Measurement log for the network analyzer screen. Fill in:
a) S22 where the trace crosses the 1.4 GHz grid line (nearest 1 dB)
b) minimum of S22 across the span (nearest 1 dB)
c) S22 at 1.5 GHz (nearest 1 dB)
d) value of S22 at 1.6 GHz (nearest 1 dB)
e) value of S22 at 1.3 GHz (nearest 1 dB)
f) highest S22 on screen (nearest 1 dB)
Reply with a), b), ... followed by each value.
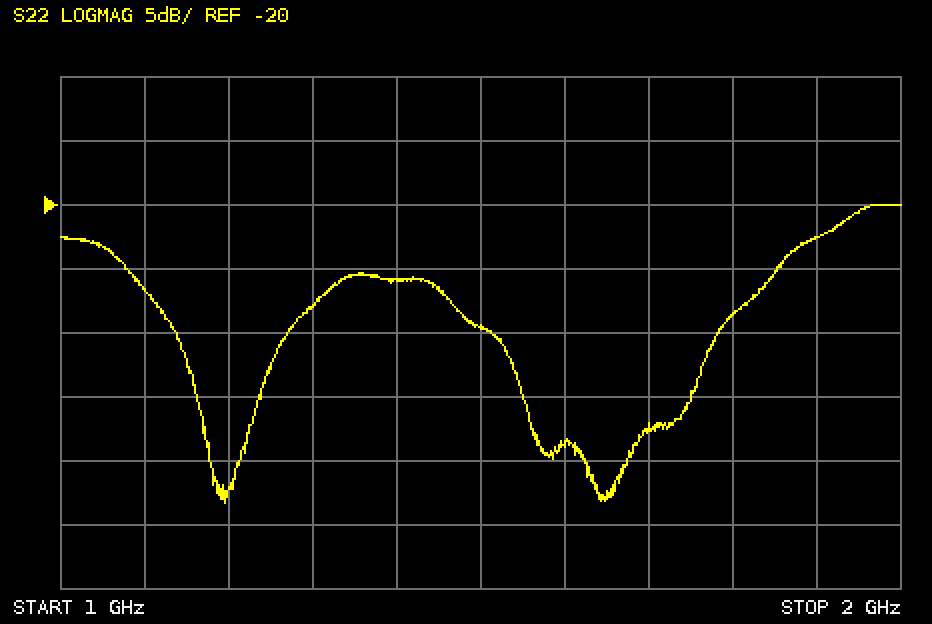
a) -26 dB
b) -43 dB
c) -30 dB
d) -39 dB
e) -28 dB
f) -20 dB
